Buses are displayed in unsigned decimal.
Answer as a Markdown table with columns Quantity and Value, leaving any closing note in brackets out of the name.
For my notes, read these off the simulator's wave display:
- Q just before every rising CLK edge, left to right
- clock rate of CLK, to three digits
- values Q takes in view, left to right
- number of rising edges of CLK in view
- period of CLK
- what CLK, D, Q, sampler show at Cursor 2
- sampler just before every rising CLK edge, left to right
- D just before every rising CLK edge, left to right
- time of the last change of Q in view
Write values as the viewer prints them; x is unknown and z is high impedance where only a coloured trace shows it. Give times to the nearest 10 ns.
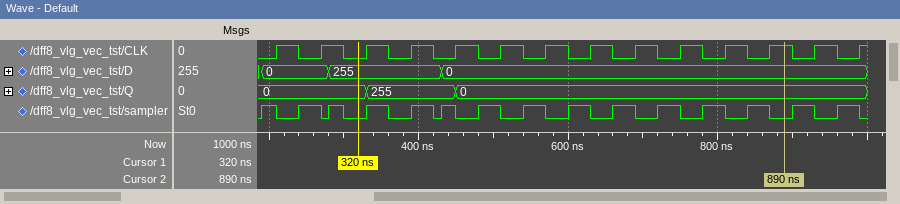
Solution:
| Quantity | Value |
|---|---|
| Q just before every rising CLK edge, left to right | 0, 0, 0, 255, 255, 0, 0, 0, 0, 0, 0, 0, 0, 0 |
| clock rate of CLK, to three digits | 16.7 MHz |
| values Q takes in view, left to right | 0, 255, 0 |
| number of rising edges of CLK in view | 14 |
| period of CLK | 60 ns |
| what CLK, D, Q, sampler show at Cursor 2 | CLK=1, D=0, Q=0, sampler=0 |
| sampler just before every rising CLK edge, left to right | 1 1 0 0 1 1 1 1 1 1 1 1 1 1 |
| D just before every rising CLK edge, left to right | 0, 0, 255, 255, 0, 0, 0, 0, 0, 0, 0, 0, 0, 0 |
| time of the last change of Q in view | 450 ns |
